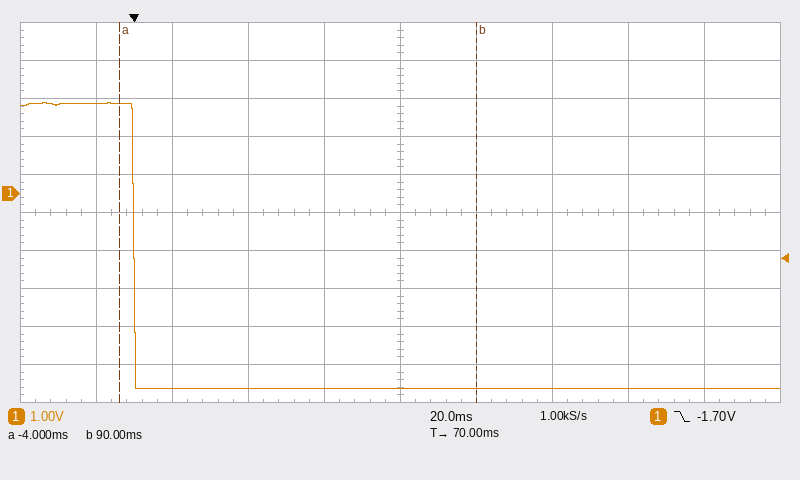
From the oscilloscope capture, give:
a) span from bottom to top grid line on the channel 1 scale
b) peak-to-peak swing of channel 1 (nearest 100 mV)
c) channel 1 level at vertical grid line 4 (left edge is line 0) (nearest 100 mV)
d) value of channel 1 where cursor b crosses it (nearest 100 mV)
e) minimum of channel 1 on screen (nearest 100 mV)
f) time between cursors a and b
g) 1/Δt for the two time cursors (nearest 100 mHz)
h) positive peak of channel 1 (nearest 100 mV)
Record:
10 V
7.5 V
-5.1 V
-5.1 V
-5.1 V
94 ms
10.6 Hz
2.4 V
